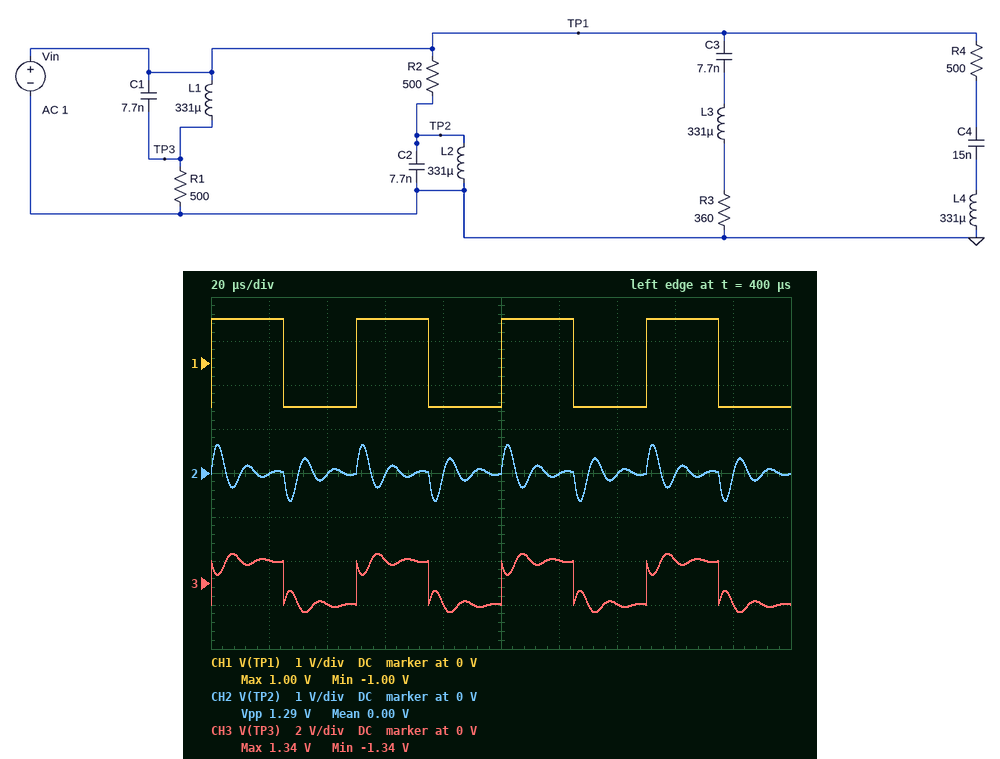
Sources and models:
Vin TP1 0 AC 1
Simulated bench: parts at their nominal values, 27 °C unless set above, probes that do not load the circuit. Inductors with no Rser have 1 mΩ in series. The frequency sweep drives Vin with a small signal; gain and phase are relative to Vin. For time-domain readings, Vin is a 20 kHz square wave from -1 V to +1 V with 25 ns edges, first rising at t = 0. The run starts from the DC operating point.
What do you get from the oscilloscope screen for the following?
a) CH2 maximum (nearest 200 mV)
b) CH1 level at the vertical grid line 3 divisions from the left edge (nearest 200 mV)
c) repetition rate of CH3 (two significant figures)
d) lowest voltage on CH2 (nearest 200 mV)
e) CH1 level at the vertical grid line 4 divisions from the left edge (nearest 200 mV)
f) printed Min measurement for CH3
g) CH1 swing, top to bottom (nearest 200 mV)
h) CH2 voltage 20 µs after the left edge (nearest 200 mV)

600 mV
1.0 V
20 kHz
-600 mV
-1.0 V
-1.34 V
2.0 V
0 V
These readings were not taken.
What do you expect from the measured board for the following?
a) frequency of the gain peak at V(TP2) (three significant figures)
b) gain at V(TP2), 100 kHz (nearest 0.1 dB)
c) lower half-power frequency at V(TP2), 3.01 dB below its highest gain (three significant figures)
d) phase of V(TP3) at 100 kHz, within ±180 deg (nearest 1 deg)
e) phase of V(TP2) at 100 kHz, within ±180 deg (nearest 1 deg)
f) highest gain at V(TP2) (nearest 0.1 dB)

99.7 kHz
0 dB
81.1 kHz
89 deg
-1 deg
0 dB
